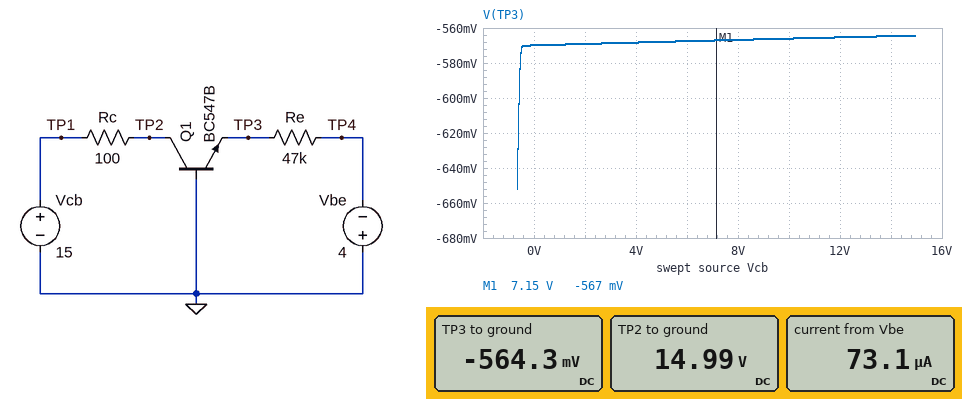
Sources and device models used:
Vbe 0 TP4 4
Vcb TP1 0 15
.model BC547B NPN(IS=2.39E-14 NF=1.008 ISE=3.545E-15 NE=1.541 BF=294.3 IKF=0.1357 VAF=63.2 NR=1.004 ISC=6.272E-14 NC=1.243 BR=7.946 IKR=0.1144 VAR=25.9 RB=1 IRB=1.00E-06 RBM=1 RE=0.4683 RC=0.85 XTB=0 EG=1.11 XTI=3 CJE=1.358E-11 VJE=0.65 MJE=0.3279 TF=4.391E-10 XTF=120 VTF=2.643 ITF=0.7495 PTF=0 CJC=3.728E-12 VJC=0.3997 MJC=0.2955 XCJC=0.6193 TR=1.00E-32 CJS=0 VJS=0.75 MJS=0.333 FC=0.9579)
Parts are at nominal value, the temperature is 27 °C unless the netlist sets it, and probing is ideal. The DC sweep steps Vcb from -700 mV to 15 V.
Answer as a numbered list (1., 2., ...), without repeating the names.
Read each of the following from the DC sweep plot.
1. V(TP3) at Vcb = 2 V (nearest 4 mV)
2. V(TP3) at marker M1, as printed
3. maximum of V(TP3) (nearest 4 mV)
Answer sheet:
1. -568 mV
2. -567 mV
3. -564 mV
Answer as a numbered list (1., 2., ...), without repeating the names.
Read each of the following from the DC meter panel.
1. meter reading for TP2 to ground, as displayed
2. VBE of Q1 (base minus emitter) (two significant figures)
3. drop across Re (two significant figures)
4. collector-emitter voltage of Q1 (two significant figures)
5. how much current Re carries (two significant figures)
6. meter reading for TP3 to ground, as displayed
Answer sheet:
1. 14.99 V
2. 560 mV
3. 3.4 V
4. 16 V
5. 73 µA
6. -564.3 mV
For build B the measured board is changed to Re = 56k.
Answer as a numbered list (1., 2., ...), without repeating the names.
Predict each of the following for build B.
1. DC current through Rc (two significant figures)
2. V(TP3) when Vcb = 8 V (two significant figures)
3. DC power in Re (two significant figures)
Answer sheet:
1. 61 µA
2. -560 mV
3. 210 µW
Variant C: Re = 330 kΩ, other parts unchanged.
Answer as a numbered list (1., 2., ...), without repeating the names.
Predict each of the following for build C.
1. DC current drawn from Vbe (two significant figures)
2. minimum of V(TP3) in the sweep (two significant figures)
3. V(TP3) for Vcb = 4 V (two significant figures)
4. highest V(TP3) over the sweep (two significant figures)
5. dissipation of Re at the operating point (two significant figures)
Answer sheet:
1. 11 µA
2. -660 mV
3. -520 mV
4. -510 mV
5. 37 µW
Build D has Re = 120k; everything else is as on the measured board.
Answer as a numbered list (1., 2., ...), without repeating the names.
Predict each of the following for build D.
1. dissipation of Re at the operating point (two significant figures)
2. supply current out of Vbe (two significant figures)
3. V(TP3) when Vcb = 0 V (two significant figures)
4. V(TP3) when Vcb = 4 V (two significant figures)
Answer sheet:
1. 100 µW
2. 29 µA
3. -550 mV
4. -540 mV
